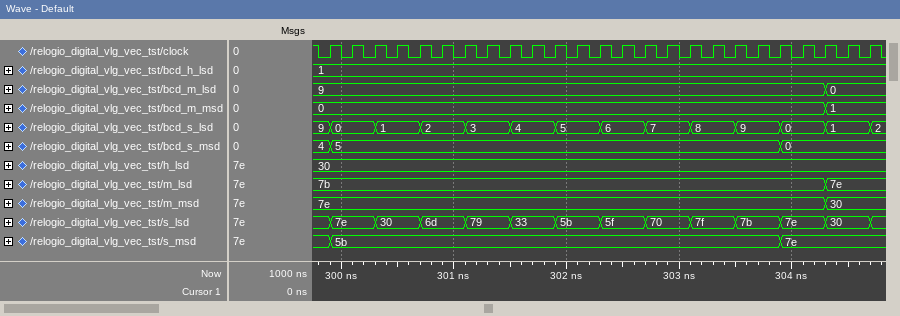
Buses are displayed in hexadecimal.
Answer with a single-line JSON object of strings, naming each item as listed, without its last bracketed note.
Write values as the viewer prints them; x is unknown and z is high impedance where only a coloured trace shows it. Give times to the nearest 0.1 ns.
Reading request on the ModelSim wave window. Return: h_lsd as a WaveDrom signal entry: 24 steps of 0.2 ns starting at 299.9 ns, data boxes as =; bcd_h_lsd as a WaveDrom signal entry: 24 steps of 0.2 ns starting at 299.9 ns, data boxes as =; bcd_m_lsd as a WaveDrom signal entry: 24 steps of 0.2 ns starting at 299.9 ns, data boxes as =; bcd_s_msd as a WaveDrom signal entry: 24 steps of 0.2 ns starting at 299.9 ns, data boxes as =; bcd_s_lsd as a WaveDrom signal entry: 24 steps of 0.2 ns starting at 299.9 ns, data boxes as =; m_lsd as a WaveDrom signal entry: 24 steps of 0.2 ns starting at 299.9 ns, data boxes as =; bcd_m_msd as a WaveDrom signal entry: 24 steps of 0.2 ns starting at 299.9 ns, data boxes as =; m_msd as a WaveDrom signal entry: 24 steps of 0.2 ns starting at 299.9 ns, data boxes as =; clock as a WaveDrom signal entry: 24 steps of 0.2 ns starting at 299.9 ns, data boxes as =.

{"h_lsd as a WaveDrom signal entry: 24 steps of 0.2 ns starting at 299.9 ns, data boxes as =": "{name: 'h_lsd', wave: '=.......................', data: '30'}", "bcd_h_lsd as a WaveDrom signal entry: 24 steps of 0.2 ns starting at 299.9 ns, data boxes as =": "{name: 'bcd_h_lsd', wave: '=.......................', data: '1'}", "bcd_m_lsd as a WaveDrom signal entry: 24 steps of 0.2 ns starting at 299.9 ns, data boxes as =": "{name: 'bcd_m_lsd', wave: '=.....................=.', data: '9 0'}", "bcd_s_msd as a WaveDrom signal entry: 24 steps of 0.2 ns starting at 299.9 ns, data boxes as =": "{name: 'bcd_s_msd', wave: '=...................=...', data: '5 0'}", "bcd_s_lsd as a WaveDrom signal entry: 24 steps of 0.2 ns starting at 299.9 ns, data boxes as =": "{name: 'bcd_s_lsd', wave: '=.=.=.=.=.=.=.=.=.=.=.=.', data: '0 1 2 3 4 5 6 7 8 9 0 1'}", "m_lsd as a WaveDrom signal entry: 24 steps of 0.2 ns starting at 299.9 ns, data boxes as =": "{name: 'm_lsd', wave: '=.....................=.', data: '7b 7e'}", "bcd_m_msd as a WaveDrom signal entry: 24 steps of 0.2 ns starting at 299.9 ns, data boxes as =": "{name: 'bcd_m_msd', wave: '=.....................=.', data: '0 1'}", "m_msd as a WaveDrom signal entry: 24 steps of 0.2 ns starting at 299.9 ns, data boxes as =": "{name: 'm_msd', wave: '=.....................=.', data: '7e 30'}", "clock as a WaveDrom signal entry: 24 steps of 0.2 ns starting at 299.9 ns, data boxes as =": "{name: 'clock', wave: 'p.......................'}"}
